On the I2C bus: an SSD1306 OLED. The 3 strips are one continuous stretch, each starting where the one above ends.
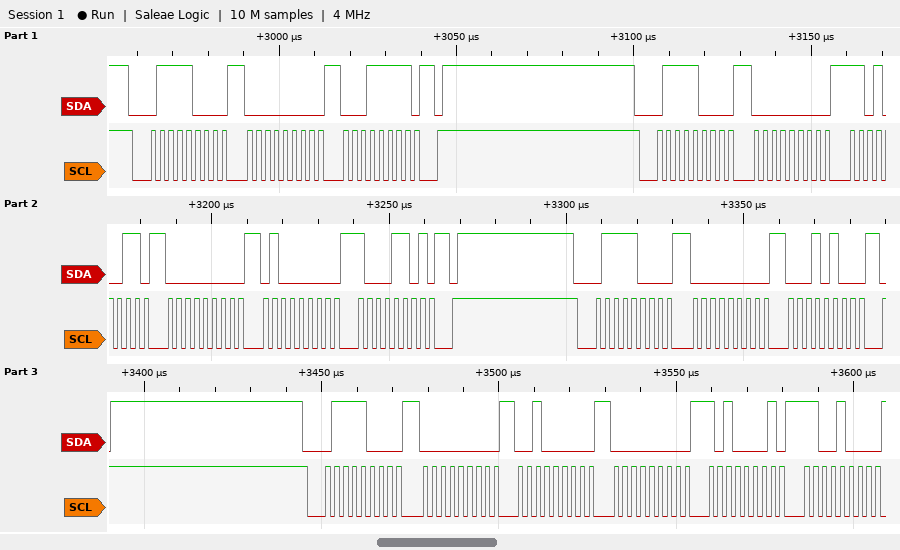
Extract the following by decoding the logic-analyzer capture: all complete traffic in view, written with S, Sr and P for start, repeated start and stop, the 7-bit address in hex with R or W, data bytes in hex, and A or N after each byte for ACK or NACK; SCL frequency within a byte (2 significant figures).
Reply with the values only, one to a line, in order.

S 3CW A 00 A 1F A P S 3CW A 00 A D3 A 00 A 40 A 8D A P S 3CW A 00 A 14 A P S 3CW A 00 A 20 A 00 A A1 A C8 A
400 kHz
